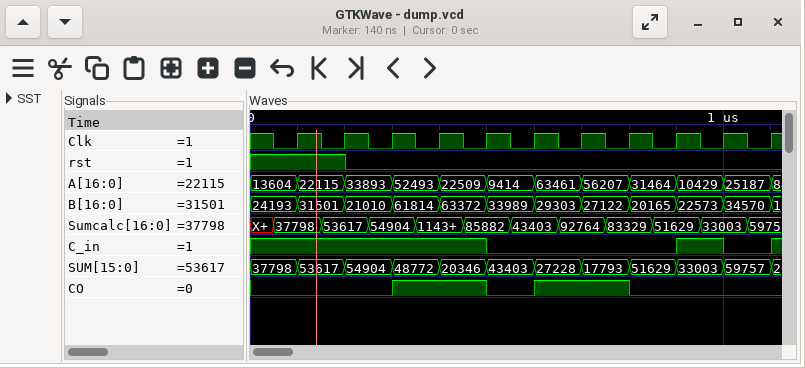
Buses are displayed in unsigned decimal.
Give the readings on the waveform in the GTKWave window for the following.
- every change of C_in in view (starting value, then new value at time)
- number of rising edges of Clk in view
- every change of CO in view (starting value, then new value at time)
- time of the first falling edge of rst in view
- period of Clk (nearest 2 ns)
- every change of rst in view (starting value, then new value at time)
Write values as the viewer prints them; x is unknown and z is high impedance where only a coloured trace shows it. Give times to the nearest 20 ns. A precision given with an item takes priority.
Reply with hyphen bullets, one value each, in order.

- 1, 0 at 500 ns, 1 at 900 ns, 0 at 1000 ns, 1 at 1100 ns
- 11
- 0, 1 at 300 ns, 0 at 500 ns, 1 at 600 ns, 0 at 800 ns
- 200 ns
- 100 ns
- 1, 0 at 200 ns
